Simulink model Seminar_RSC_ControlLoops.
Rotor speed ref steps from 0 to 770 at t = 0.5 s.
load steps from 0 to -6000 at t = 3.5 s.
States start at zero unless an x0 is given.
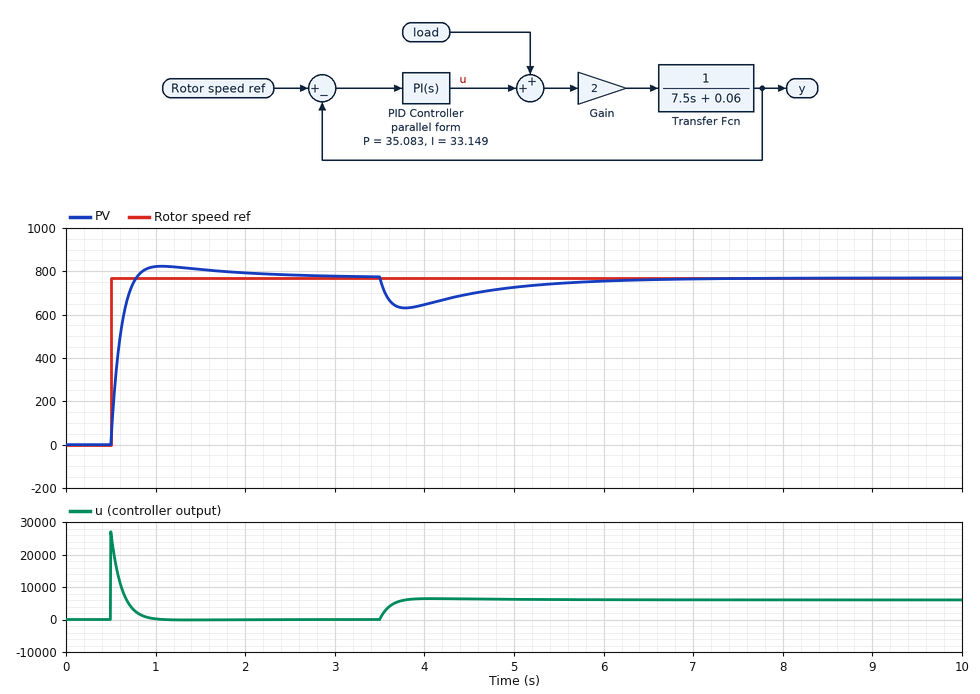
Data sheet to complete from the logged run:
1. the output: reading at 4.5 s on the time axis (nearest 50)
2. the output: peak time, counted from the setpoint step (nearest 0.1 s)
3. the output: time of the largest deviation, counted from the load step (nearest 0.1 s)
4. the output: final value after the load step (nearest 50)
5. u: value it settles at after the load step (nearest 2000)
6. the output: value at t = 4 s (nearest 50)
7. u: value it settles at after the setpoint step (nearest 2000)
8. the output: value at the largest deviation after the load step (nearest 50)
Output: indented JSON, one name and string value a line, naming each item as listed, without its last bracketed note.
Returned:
{
  "the output: reading at 4.5 s on the time axis": "700",
  "the output: peak time, counted from the setpoint step": "0.6 s",
  "the output: time of the largest deviation, counted from the load step": "0.3 s",
  "the output: final value after the load step": "750",
  "u: value it settles at after the load step": "6000",
  "the output: value at t = 4 s": "650",
  "u: value it settles at after the setpoint step": "0",
  "the output: value at the largest deviation after the load step": "650"
}
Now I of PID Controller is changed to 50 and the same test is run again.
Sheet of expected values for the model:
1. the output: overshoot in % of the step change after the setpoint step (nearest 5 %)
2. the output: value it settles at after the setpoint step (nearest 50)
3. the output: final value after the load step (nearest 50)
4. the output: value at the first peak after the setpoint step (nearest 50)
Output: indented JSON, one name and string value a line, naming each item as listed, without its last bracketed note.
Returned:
{
  "the output: overshoot in % of the step change after the setpoint step": "10 %",
  "the output: value it settles at after the setpoint step": "750",
  "the output: final value after the load step": "750",
  "the output: value at the first peak after the setpoint step": "850"
}
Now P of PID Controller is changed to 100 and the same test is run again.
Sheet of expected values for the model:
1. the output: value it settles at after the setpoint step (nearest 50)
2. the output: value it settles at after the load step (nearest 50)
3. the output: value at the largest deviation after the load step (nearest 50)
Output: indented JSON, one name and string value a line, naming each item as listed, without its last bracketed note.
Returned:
{
  "the output: value it settles at after the setpoint step": "750",
  "the output: value it settles at after the load step": "750",
  "the output: value at the largest deviation after the load step": "700"
}
